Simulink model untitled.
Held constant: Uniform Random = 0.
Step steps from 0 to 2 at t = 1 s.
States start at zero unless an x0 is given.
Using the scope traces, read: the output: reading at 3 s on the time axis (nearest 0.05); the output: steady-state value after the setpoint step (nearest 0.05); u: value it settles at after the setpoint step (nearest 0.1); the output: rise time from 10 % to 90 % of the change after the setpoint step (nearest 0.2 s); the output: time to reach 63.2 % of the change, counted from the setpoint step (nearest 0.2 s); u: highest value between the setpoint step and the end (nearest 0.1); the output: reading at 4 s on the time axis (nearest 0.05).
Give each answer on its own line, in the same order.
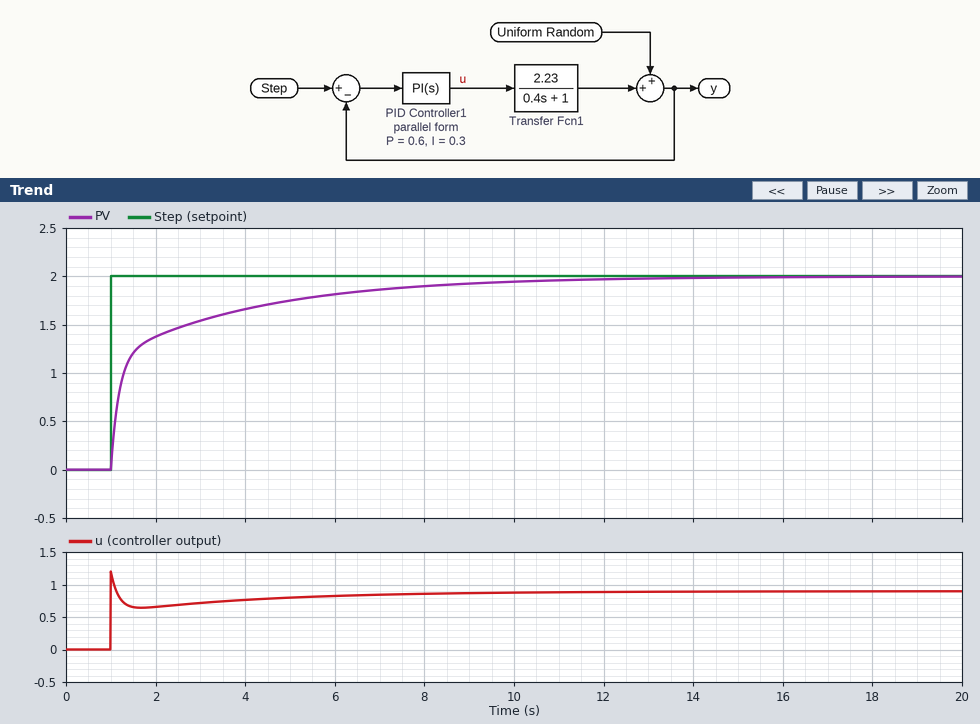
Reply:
1.55
2.00
0.9
4.8 s
0.6 s
1.2
1.65
